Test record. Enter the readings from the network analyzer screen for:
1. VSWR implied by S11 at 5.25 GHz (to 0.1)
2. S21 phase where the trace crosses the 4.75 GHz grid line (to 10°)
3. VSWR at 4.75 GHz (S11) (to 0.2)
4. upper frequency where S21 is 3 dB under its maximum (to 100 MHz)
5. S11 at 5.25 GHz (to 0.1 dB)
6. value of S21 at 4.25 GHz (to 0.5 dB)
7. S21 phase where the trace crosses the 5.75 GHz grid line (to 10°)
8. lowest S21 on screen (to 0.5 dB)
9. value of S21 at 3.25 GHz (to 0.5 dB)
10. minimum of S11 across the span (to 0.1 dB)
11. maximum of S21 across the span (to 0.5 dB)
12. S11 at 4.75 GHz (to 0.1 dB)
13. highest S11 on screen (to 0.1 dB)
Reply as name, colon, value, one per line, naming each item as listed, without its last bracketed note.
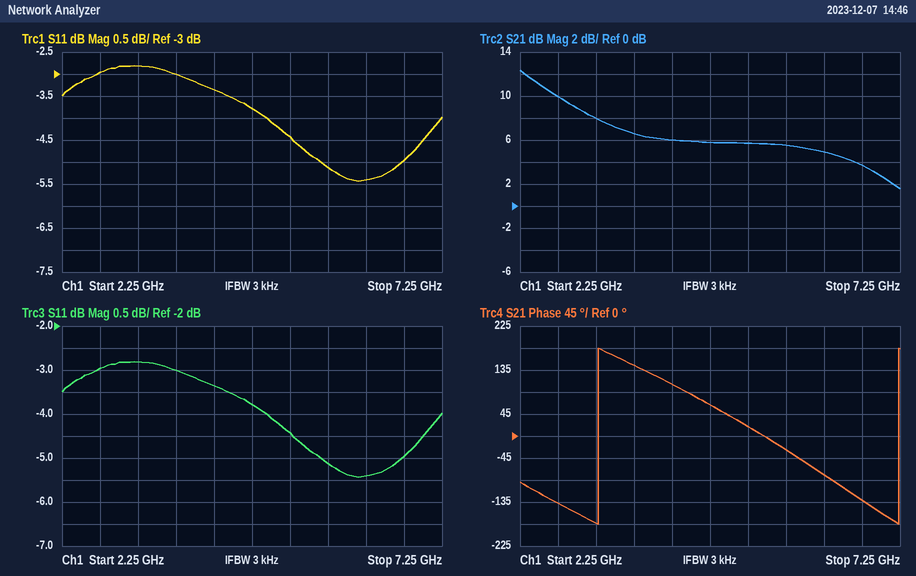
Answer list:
VSWR implied by S11 at 5.25 GHz: 4.0
S21 phase where the trace crosses the 4.75 GHz grid line: 60°
VSWR at 4.75 GHz (S11): 4.6
upper frequency where S21 is 3 dB under its maximum: 2.9 GHz
S11 at 5.25 GHz: -4.4 dB
value of S21 at 4.25 GHz: 6.0 dB
S21 phase where the trace crosses the 5.75 GHz grid line: -30°
lowest S21 on screen: 1.5 dB
value of S21 at 3.25 GHz: 8.0 dB
minimum of S11 across the span: -5.4 dB
maximum of S21 across the span: 12.5 dB
S11 at 4.75 GHz: -3.8 dB
highest S11 on screen: -2.8 dB
